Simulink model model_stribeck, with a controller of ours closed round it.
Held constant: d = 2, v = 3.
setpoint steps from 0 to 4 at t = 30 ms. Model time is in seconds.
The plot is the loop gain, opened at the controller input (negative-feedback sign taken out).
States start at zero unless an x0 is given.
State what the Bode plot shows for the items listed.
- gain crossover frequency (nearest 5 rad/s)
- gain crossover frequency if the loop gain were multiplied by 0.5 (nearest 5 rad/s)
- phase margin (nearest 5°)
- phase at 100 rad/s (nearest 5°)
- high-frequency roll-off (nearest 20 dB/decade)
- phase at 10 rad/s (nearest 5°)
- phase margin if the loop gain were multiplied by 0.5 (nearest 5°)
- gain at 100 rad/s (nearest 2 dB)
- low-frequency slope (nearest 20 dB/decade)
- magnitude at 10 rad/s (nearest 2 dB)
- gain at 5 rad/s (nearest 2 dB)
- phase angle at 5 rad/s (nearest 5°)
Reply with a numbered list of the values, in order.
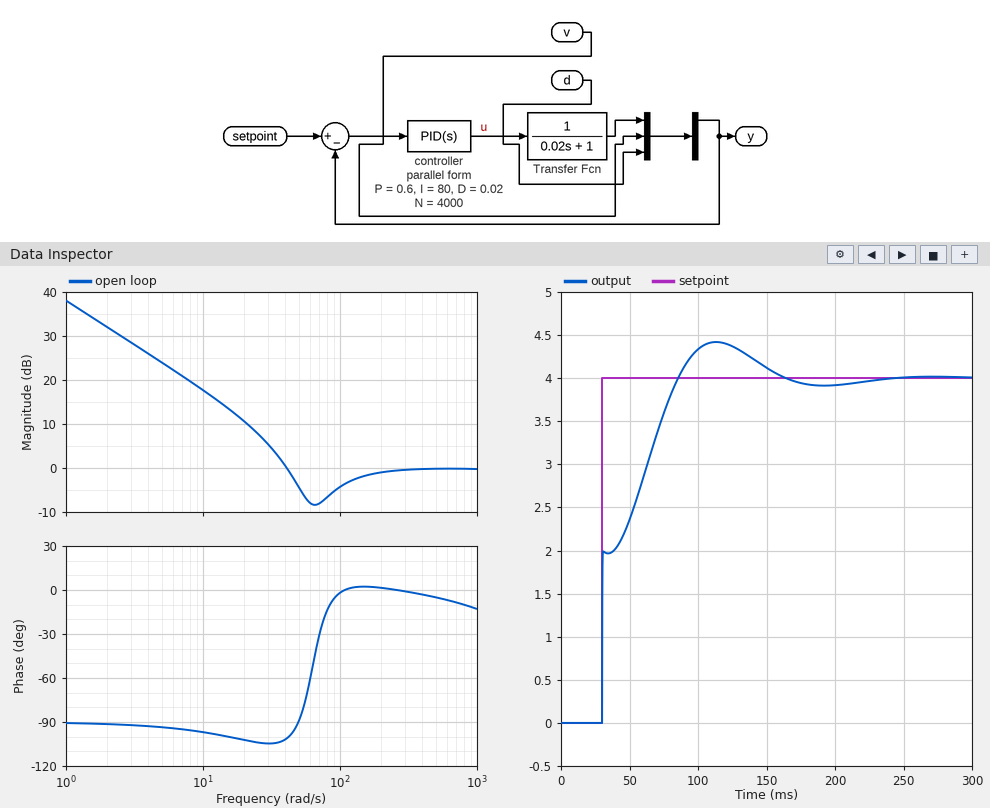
1. 40 rad/s
2. 30 rad/s
3. 80°
4. 0°
5. 0 dB/decade
6. -95°
7. 75°
8. -4 dB
9. -20 dB/decade
10. 18 dB
11. 24 dB
12. -95°
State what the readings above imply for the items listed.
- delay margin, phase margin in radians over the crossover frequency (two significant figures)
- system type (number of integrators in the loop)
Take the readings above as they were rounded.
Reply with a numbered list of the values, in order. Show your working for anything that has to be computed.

1. 80 × π / 180 / 40 = 0.035 s
2. 1
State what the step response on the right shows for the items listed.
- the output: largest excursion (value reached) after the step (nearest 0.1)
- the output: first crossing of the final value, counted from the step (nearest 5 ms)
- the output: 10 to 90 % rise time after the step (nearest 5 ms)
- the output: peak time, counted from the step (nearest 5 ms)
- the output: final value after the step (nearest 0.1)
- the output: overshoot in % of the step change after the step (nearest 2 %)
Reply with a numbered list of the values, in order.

1. 4.4
2. 55 ms
3. 45 ms
4. 85 ms
5. 4.0
6. 10 %
